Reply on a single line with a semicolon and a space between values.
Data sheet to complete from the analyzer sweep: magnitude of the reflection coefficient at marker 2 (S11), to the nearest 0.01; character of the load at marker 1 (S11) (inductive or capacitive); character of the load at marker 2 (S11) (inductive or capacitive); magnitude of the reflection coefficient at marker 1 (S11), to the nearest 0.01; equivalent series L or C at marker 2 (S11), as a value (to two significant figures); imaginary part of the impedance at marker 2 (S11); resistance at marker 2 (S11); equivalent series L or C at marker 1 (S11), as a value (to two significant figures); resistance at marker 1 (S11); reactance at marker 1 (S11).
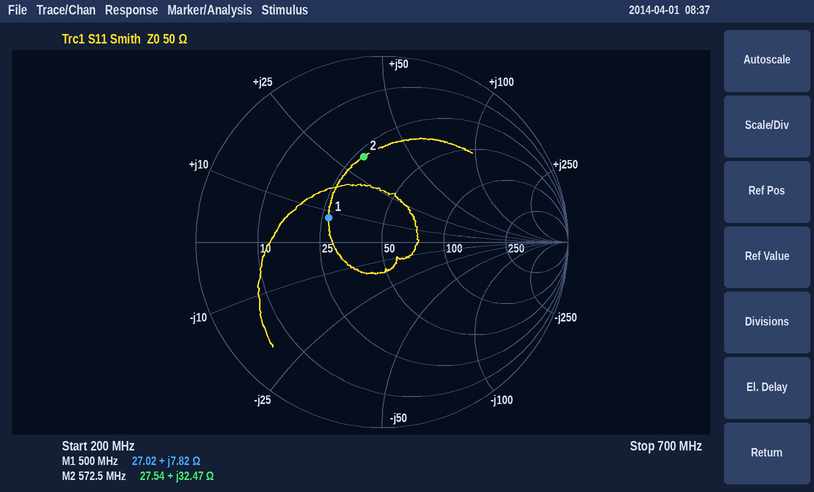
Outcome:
0.47; inductive; inductive; 0.31; 9.0 nH; +32.47 Ω; 27.54 Ω; 2.5 nH; 27.02 Ω; +7.82 Ω
